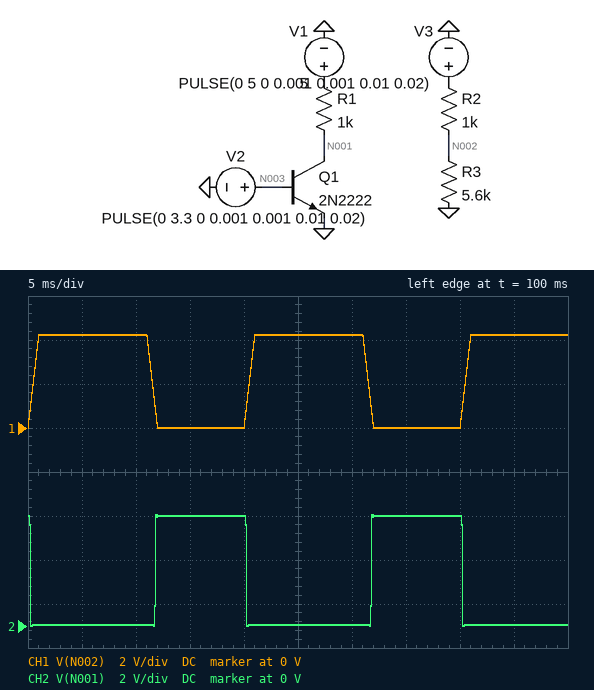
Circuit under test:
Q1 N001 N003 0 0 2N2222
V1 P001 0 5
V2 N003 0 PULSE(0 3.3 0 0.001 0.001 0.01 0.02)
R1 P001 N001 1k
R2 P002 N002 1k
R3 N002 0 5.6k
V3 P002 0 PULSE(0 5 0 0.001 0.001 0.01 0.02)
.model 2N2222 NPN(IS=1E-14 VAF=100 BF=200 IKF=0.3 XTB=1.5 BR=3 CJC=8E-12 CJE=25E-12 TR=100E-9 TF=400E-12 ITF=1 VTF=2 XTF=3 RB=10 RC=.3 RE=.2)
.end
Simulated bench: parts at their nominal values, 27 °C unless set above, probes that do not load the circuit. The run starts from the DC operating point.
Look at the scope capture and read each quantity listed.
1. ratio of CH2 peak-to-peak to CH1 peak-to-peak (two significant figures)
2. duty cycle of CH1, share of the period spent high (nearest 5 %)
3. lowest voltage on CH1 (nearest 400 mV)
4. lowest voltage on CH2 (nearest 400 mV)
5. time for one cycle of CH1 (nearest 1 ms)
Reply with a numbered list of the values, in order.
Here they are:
1. 1.2
2. 55 %
3. 0 V
4. 0 V
5. 20 ms
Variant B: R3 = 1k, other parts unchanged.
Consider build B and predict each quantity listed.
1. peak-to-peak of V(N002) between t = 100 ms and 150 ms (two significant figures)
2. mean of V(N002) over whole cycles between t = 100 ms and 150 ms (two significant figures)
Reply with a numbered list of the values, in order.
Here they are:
1. 2.5 V
2. 1.4 V
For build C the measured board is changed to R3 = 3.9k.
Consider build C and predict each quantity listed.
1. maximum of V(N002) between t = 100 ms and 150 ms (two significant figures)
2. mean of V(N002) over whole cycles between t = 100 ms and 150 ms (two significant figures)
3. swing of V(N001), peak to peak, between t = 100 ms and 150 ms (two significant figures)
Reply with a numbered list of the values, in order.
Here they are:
1. 4.0 V
2. 2.2 V
3. 5.0 V
